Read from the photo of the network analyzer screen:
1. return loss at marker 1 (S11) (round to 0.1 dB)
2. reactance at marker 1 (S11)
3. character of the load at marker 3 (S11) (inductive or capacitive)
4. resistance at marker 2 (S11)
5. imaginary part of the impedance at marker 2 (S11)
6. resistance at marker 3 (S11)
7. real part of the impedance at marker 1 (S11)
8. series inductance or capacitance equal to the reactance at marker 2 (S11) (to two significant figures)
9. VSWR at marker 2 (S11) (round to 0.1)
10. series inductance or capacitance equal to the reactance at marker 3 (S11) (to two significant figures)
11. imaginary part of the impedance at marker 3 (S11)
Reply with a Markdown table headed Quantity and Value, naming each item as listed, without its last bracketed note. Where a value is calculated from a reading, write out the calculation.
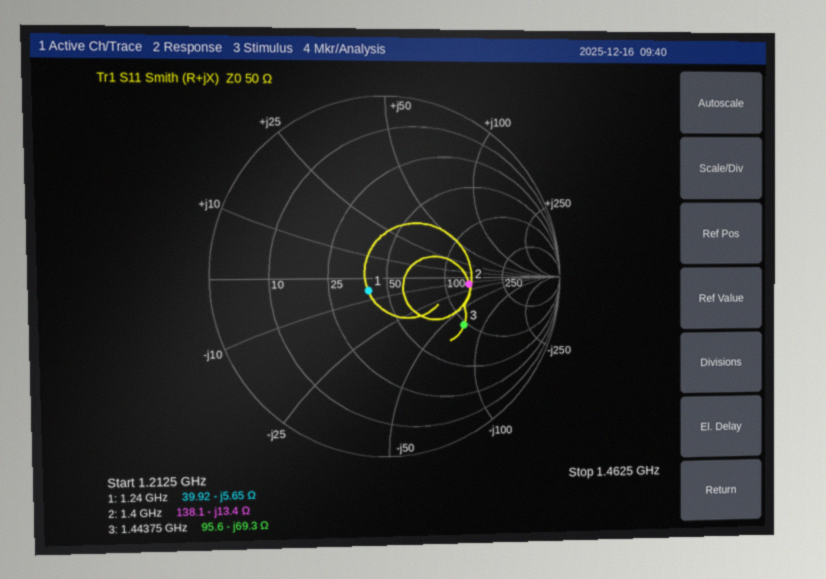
| Quantity | Value |
|---|---|
| return loss at marker 1 (S11) | 17.8 dB |
| reactance at marker 1 | -5.65 Ω |
| character of the load at marker 3 (S11) | capacitive |
| resistance at marker 2 | 138.1 Ω |
| imaginary part of the impedance at marker 2 | -13.4 Ω |
| resistance at marker 3 | 95.6 Ω |
| real part of the impedance at marker 1 | 39.92 Ω |
| series inductance or capacitance equal to the reactance at marker 2 (S11) | C = 1/(2π × 1.4 GHz × 13.4 Ω) ≈ 8.5 pF |
| VSWR at marker 2 (S11) | 2.8 |
| series inductance or capacitance equal to the reactance at marker 3 (S11) | C = 1/(2π × 1.44375 GHz × 69.3 Ω) ≈ 1.6 pF |
| imaginary part of the impedance at marker 3 | -69.3 Ω |
